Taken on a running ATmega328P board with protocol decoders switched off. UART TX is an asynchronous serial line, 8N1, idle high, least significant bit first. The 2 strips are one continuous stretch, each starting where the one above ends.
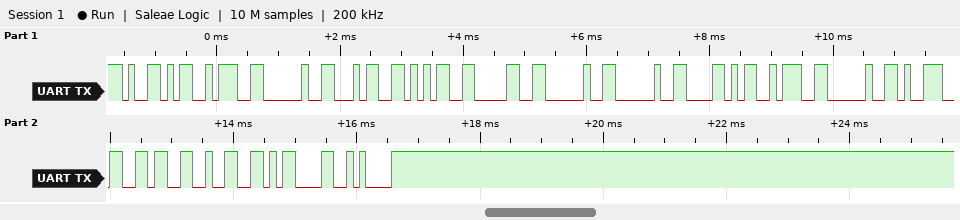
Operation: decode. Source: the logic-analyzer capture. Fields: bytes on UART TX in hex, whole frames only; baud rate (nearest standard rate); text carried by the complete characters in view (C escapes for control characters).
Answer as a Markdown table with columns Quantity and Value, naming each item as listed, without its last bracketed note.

| Quantity | Value |
|---|---|
| bytes on UART TX in hex, whole frames only | 59 3A 20 34 35 30 20 20 58 3A 20 39 36 32 0D 0A |
| baud rate | 9600 baud |
| text carried by the complete characters in view | "Y: 450  X: 962\r\n" |
